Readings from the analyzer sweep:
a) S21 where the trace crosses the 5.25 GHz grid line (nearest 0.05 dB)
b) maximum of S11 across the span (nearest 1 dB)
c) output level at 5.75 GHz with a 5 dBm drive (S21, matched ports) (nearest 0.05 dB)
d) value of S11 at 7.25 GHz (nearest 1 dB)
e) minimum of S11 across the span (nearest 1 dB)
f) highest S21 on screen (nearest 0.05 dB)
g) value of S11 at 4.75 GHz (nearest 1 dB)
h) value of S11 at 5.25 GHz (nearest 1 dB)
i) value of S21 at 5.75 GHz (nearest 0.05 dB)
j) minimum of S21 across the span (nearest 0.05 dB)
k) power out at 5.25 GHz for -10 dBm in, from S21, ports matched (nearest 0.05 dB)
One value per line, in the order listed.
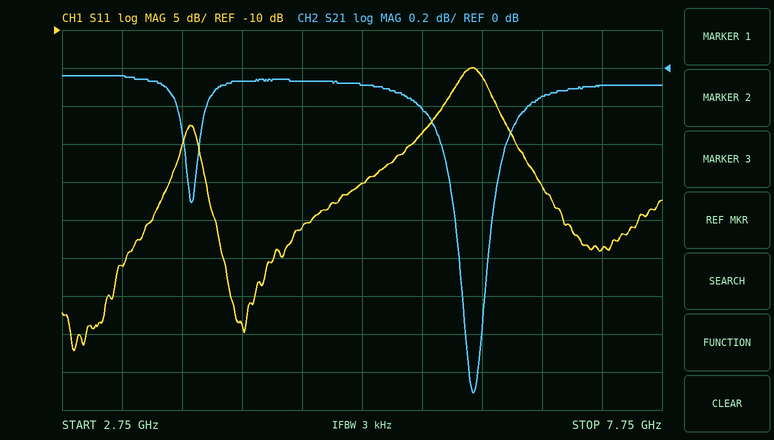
-0.10 dB
-15 dB
4.80 dBm
-39 dB
-52 dB
-0.05 dB
-36 dB
-30 dB
-0.20 dB
-1.70 dB
-10.10 dBm
